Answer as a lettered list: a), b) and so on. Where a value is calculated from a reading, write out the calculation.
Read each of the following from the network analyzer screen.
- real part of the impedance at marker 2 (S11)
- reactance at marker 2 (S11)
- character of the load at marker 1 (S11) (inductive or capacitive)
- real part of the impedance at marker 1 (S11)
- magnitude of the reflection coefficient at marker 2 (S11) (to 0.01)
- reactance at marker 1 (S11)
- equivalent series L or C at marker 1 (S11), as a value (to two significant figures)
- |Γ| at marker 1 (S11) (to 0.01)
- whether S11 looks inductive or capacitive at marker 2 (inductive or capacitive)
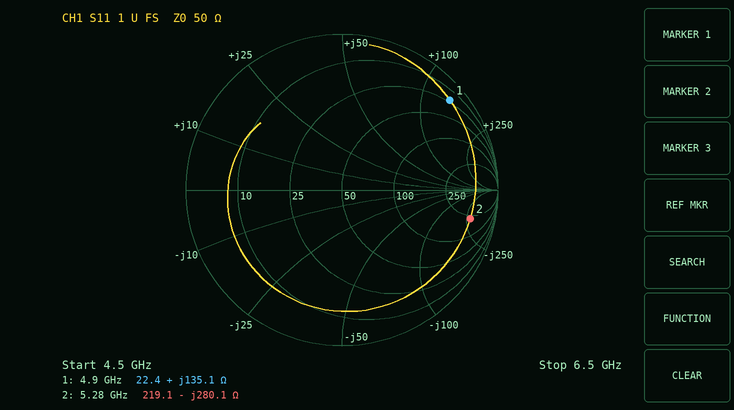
a) 219.1 Ω
b) -280.1 Ω
c) inductive
d) 22.4 Ω
e) 0.84
f) +135.1 Ω
g) L = 135.1 Ω/(2π × 4.9 GHz) ≈ 4.4 nH
h) 0.90
i) capacitive
